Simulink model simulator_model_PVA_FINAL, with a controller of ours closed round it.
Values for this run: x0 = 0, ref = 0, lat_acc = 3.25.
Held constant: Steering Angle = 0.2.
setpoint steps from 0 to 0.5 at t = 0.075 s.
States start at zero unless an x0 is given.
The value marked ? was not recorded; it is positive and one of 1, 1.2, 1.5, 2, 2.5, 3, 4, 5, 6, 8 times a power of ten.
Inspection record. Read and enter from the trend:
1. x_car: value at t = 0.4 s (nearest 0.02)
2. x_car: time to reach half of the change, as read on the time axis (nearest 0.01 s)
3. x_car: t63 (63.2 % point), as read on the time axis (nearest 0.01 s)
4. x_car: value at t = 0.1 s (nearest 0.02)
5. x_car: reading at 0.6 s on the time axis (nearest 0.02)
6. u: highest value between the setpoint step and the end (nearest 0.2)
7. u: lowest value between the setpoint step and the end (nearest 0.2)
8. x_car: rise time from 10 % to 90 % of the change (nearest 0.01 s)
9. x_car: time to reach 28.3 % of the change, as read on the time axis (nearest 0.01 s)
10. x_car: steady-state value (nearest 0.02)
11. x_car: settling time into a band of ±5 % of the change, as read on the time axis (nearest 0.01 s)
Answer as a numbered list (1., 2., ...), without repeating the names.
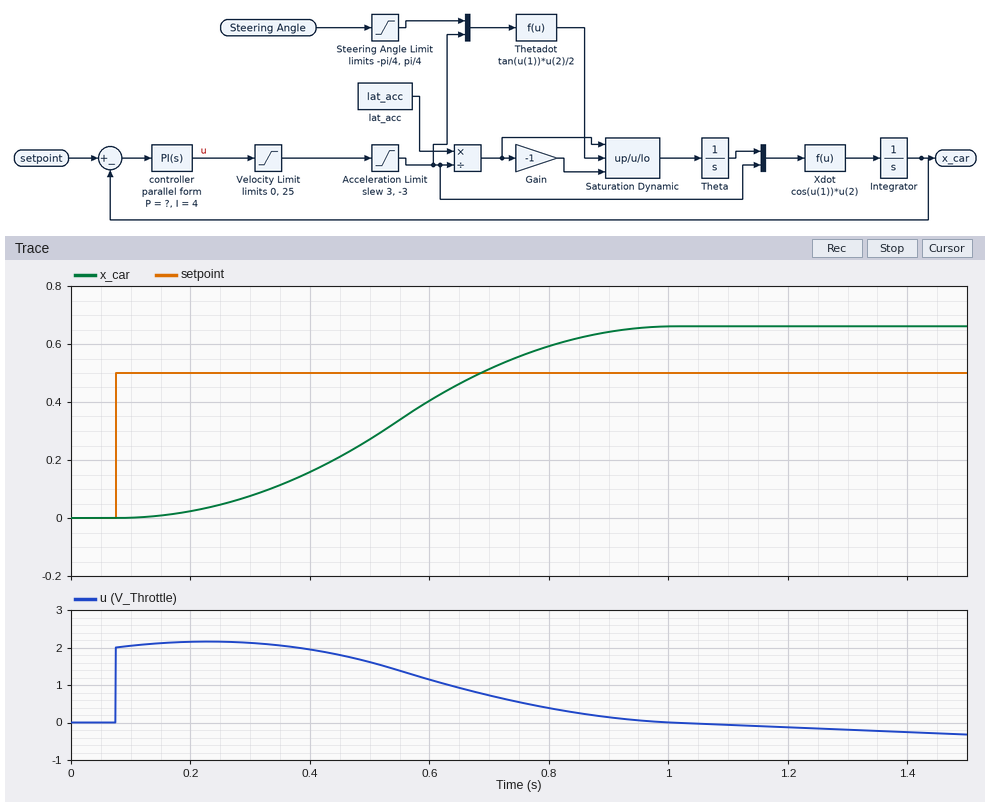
1. 0.16
2. 0.54 s
3. 0.61 s
4. 0.00
5. 0.40
6. 2.2
7. -0.4
8. 0.52 s
9. 0.43 s
10. 0.66
11. 0.86 s
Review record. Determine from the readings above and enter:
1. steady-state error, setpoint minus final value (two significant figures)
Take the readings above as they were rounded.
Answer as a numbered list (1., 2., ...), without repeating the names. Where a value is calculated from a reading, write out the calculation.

1. 0.5 - 0.66 = -0.16
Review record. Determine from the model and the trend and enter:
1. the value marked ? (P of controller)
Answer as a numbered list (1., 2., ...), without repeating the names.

1. 4
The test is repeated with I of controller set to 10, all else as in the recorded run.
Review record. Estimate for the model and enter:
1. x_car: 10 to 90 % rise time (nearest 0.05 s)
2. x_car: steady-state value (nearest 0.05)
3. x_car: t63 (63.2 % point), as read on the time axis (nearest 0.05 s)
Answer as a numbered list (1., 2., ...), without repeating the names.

1. 0.65 s
2. 1.05
3. 0.75 s
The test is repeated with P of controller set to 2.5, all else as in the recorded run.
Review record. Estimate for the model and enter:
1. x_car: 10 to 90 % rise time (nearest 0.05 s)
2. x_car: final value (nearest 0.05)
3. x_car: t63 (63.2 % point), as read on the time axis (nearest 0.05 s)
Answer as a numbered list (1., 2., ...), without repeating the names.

1. 0.65 s
2. 0.70
3. 0.65 s
